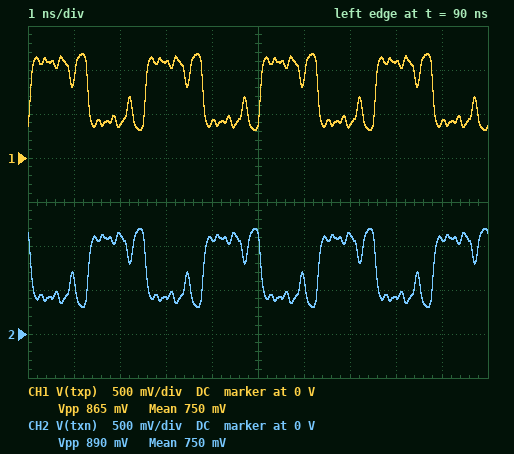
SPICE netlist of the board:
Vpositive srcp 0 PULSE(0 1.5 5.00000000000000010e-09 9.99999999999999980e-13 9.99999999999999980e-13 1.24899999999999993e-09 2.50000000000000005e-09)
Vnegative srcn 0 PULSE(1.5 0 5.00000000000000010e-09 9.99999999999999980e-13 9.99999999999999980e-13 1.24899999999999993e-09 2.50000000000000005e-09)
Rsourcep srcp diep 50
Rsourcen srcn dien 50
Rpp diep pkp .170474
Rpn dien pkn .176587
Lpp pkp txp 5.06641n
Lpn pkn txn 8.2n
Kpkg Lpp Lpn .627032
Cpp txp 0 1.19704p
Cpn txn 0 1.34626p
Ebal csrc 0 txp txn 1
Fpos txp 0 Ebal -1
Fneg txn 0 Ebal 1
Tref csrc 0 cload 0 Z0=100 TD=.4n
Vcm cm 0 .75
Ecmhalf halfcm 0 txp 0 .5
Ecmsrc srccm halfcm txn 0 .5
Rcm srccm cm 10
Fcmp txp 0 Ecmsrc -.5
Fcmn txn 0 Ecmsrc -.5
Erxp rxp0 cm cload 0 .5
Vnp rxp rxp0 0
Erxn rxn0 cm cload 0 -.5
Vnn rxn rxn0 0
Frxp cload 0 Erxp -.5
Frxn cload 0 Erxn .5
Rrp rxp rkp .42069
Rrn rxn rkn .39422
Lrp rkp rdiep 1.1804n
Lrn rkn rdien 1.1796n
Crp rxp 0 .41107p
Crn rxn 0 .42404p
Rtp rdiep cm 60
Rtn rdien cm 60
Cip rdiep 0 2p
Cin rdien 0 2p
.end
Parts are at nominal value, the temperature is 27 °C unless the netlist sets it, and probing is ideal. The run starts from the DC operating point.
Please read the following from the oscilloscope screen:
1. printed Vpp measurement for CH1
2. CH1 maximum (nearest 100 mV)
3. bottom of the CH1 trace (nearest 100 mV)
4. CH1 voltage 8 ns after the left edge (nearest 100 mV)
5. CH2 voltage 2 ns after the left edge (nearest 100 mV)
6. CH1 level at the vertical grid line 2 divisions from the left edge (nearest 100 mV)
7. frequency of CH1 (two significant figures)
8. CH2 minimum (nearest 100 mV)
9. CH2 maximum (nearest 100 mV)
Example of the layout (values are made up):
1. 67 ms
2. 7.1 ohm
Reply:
1. 865 mV
2. 1.2 V
3. 300 mV
4. 1.1 V
5. 1.1 V
6. 400 mV
7. 400 MHz
8. 300 mV
9. 1.2 V
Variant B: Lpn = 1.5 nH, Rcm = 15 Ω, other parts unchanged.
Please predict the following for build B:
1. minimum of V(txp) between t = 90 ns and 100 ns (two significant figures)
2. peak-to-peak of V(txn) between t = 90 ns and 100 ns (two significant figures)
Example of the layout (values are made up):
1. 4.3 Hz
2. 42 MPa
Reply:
1. 310 mV
2. 830 mV
